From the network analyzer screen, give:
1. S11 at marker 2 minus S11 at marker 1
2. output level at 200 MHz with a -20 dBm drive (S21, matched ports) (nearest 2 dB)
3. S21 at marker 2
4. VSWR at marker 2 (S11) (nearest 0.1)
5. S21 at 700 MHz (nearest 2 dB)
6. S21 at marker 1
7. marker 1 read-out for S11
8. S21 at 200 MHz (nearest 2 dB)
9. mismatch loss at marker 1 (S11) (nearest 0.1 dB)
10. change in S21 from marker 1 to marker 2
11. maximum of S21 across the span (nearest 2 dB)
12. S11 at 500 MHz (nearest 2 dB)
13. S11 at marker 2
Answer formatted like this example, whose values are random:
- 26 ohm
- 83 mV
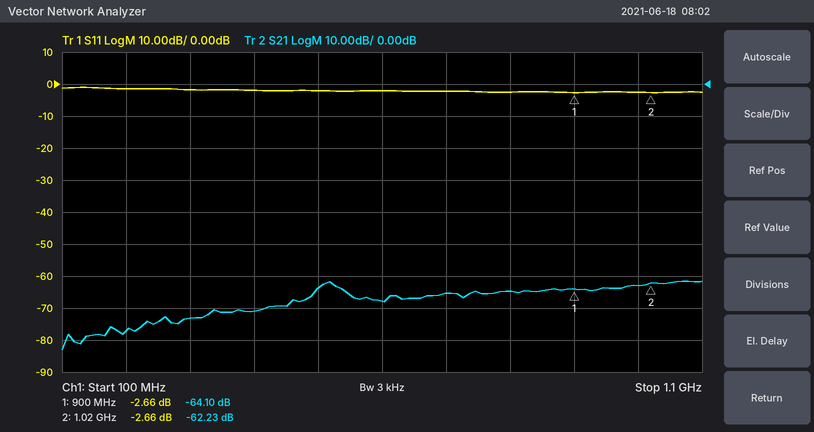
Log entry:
- 0.00 dB
- -98 dBm
- -62.23 dB
- 6.6
- -66 dB
- -64.10 dB
- -2.66 dB
- -78 dB
- 3.4 dB
- 1.87 dB
- -62 dB
- -2 dB
- -2.66 dB
